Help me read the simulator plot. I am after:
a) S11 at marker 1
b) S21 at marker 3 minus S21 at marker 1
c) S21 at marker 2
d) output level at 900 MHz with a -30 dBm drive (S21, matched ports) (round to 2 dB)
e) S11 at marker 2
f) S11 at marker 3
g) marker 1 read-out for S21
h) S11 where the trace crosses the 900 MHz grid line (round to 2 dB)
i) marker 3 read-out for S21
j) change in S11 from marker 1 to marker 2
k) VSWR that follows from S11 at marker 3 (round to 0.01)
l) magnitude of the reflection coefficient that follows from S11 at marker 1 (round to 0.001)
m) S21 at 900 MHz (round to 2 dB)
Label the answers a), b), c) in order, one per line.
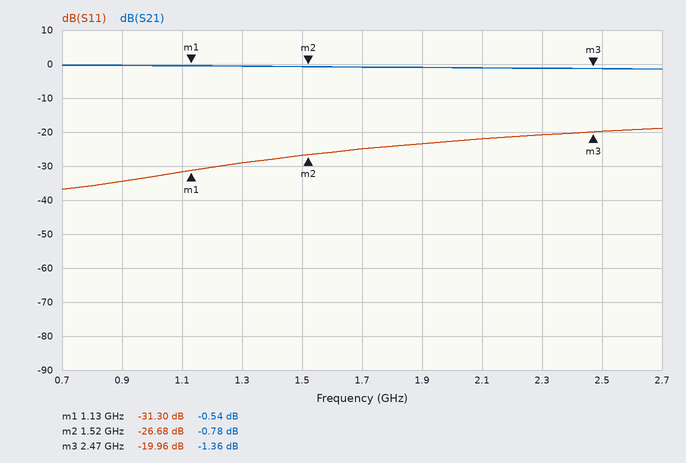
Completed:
a) -31.30 dB
b) -0.82 dB
c) -0.78 dB
d) -30 dBm
e) -26.68 dB
f) -19.96 dB
g) -0.54 dB
h) -34 dB
i) -1.36 dB
j) 4.62 dB
k) 1.22
l) 0.027
m) 0 dB
